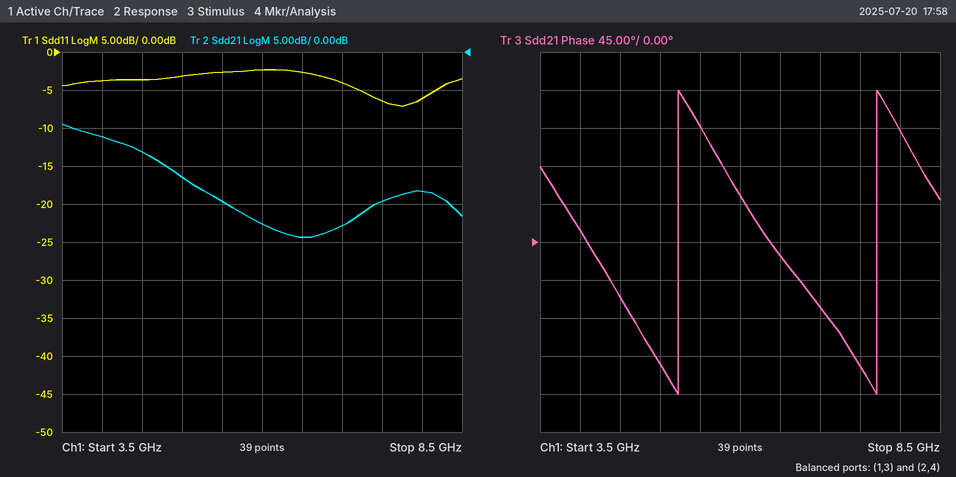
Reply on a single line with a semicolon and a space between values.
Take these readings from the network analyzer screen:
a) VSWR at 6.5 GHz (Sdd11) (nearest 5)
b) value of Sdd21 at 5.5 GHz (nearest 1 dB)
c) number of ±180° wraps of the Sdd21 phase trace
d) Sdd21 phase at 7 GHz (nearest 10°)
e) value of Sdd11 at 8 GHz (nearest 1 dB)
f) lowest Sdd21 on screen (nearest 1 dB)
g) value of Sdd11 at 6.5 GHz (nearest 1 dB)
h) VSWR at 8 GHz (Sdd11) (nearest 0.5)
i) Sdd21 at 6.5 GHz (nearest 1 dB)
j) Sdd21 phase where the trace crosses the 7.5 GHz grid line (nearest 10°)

5; -20 dB; 2; -80°; -6 dB; -24 dB; -3 dB; 3.0; -24 dB; -150°
